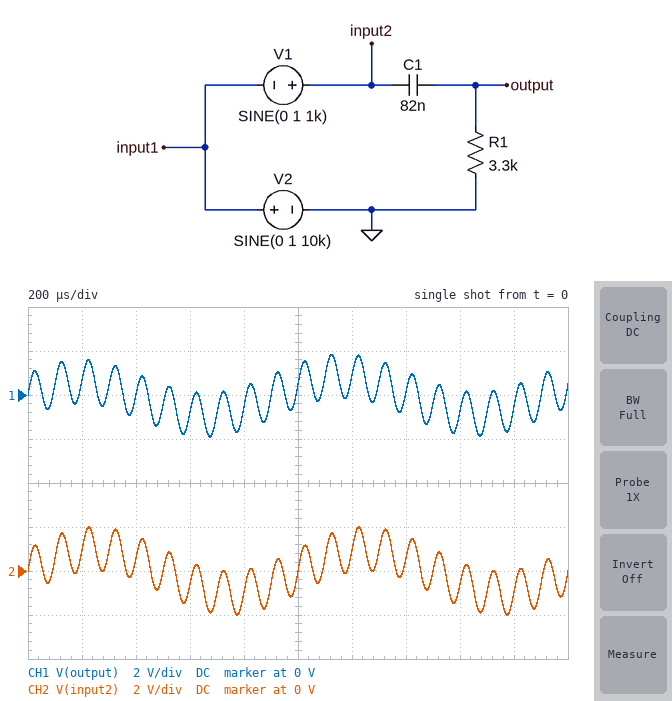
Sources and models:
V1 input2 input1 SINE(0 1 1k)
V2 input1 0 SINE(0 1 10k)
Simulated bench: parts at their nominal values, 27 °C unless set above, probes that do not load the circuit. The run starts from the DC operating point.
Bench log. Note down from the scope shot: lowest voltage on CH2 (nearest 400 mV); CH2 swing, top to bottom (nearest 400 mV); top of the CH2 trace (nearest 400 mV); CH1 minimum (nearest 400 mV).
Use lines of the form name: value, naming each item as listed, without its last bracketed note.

lowest voltage on CH2: -2.0 V
CH2 swing, top to bottom: 4.0 V
top of the CH2 trace: 2.0 V
CH1 minimum: -2.0 V
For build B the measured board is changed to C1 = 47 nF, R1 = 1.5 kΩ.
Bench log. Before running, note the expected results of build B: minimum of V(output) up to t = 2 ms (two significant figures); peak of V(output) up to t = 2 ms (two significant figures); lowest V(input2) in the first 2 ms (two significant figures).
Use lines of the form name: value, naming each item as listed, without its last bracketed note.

minimum of V(output) up to t = 2 ms: -1.4 V
peak of V(output) up to t = 2 ms: 1.4 V
lowest V(input2) in the first 2 ms: -2.0 V
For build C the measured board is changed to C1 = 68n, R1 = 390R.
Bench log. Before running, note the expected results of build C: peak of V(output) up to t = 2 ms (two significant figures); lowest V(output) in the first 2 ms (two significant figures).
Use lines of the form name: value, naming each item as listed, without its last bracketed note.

peak of V(output) up to t = 2 ms: 1.0 V
lowest V(output) in the first 2 ms: -1.0 V
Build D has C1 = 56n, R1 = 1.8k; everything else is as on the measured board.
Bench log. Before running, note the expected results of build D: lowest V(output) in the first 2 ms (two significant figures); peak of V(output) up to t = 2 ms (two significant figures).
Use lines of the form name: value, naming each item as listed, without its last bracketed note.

lowest V(output) in the first 2 ms: -1.5 V
peak of V(output) up to t = 2 ms: 1.5 V
